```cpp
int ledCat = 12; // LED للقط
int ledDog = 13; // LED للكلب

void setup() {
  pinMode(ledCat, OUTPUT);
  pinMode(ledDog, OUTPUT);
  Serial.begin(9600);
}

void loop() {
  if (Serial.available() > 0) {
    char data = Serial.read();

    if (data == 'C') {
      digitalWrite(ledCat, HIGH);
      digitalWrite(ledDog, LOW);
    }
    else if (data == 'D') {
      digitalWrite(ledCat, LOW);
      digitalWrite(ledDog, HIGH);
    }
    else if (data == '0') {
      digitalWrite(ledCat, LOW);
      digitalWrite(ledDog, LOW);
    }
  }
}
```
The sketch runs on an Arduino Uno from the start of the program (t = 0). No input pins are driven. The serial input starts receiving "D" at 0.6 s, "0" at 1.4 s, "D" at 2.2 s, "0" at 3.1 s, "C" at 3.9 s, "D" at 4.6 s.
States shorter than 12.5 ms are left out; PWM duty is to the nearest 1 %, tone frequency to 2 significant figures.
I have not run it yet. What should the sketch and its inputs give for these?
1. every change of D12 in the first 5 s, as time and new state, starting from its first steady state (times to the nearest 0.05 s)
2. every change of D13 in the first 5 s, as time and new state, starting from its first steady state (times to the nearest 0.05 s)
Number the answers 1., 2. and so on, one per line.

1. 0 s low; 3.9 s high; 4.6 s low
2. 0 s low; 0.6 s high; 1.4 s low; 2.2 s high; 3.1 s low; 4.6 s high
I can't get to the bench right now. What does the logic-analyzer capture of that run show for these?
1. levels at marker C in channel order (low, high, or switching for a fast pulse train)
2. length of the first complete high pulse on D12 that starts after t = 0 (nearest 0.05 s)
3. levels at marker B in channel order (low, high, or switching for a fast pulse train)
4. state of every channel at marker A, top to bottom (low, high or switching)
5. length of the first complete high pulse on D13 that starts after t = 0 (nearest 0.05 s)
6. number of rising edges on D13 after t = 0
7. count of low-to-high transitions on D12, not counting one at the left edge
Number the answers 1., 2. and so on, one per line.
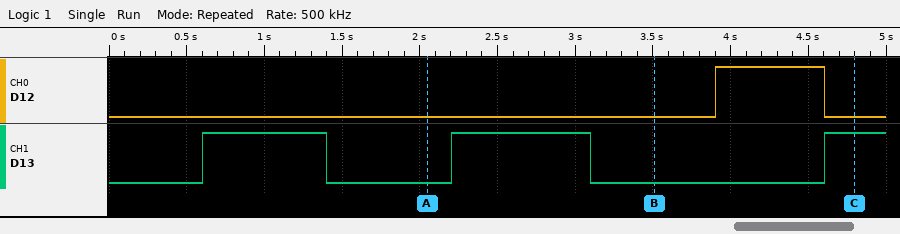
1. D12 low, D13 high
2. 0.70 s
3. D12 low, D13 low
4. D12 low, D13 low
5. 0.80 s
6. 3
7. 1
